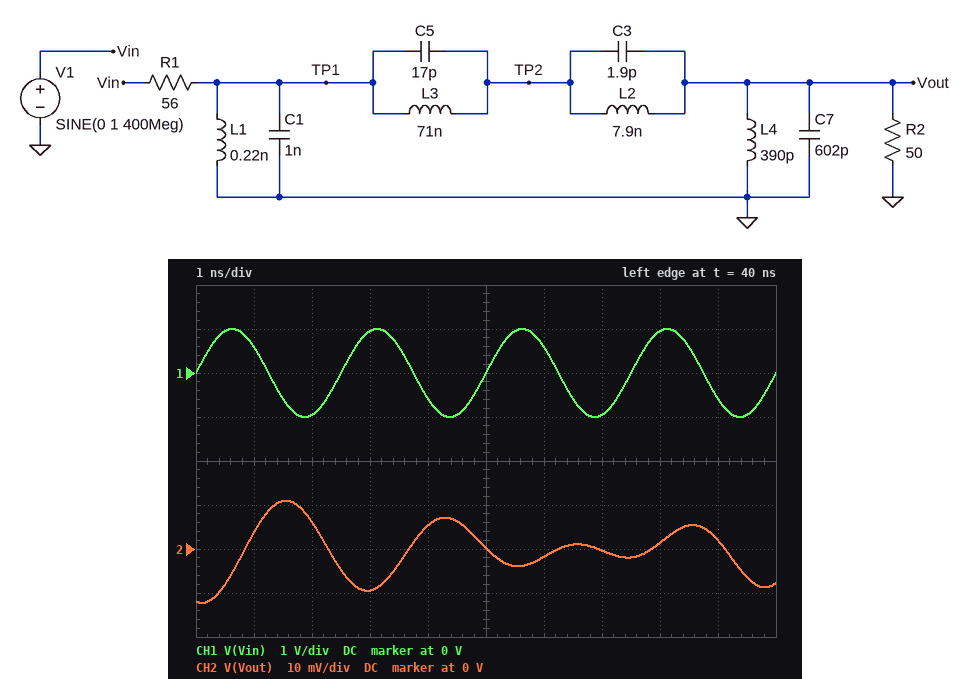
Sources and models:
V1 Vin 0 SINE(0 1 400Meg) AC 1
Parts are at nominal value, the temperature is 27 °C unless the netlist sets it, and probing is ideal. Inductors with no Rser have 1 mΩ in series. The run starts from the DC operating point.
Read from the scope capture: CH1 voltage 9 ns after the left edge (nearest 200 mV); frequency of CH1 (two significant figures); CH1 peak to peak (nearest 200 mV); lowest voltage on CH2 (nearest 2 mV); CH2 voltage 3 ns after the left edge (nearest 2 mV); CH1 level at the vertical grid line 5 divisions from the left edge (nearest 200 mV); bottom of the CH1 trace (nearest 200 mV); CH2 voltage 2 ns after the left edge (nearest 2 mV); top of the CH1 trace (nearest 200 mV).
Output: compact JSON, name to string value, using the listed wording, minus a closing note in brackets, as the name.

{"CH1 voltage 9 ns after the left edge": "-600 mV", "frequency of CH1": "400 MHz", "CH1 peak to peak": "2.0 V", "lowest voltage on CH2": "-12 mV", "CH2 voltage 3 ns after the left edge": "-10 mV", "CH1 level at the vertical grid line 5 divisions from the left edge": "0 V", "bottom of the CH1 trace": "-1.0 V", "CH2 voltage 2 ns after the left edge": "6 mV", "top of the CH1 trace": "1.0 V"}
